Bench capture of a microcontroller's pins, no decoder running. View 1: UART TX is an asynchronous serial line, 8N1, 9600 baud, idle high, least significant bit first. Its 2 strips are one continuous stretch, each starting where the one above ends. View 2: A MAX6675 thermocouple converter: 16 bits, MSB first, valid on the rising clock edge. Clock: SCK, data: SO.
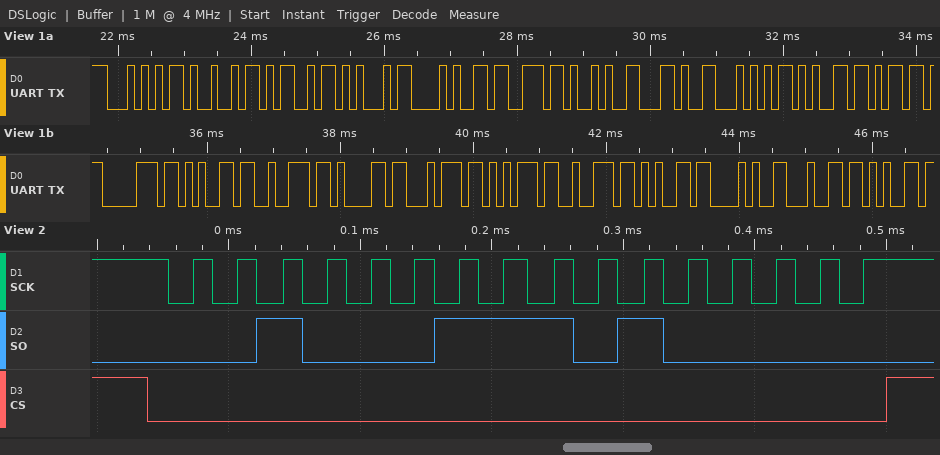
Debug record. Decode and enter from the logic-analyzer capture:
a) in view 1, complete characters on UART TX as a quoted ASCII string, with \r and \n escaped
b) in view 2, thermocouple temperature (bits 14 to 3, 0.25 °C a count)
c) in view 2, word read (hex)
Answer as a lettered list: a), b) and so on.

a) "TIME(s),Temperature(de"
b) 285.00 °C
c) 0x23A0
